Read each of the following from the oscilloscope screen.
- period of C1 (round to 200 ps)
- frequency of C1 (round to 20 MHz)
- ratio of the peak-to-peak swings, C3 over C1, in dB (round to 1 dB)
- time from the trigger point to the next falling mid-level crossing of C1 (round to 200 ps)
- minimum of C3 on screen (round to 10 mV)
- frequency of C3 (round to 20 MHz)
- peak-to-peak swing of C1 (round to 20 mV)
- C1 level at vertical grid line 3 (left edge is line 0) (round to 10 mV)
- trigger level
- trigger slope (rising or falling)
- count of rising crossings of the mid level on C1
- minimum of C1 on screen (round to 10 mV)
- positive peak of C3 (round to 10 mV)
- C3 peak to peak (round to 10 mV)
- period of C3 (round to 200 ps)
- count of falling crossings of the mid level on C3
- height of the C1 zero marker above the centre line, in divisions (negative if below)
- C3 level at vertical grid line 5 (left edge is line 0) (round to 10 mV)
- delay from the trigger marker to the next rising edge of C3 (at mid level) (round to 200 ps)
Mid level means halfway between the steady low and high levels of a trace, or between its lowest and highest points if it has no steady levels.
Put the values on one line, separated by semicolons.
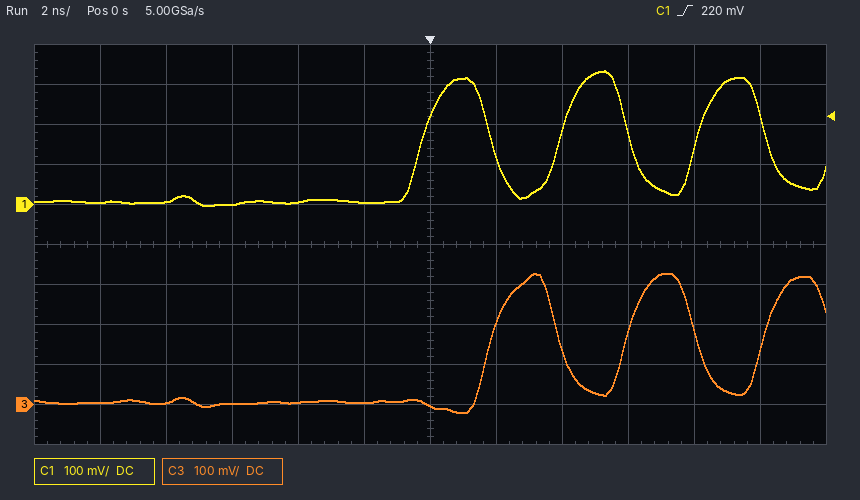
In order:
4.2 ns; 240 MHz; 0 dB; 1.8 ns; -20 mV; 240 MHz; 340 mV; 0 mV; 220 mV; rising; 3; 0 mV; 330 mV; 350 mV; 4.2 ns; 2; +1.0 div; 0 mV; 1.8 ns
